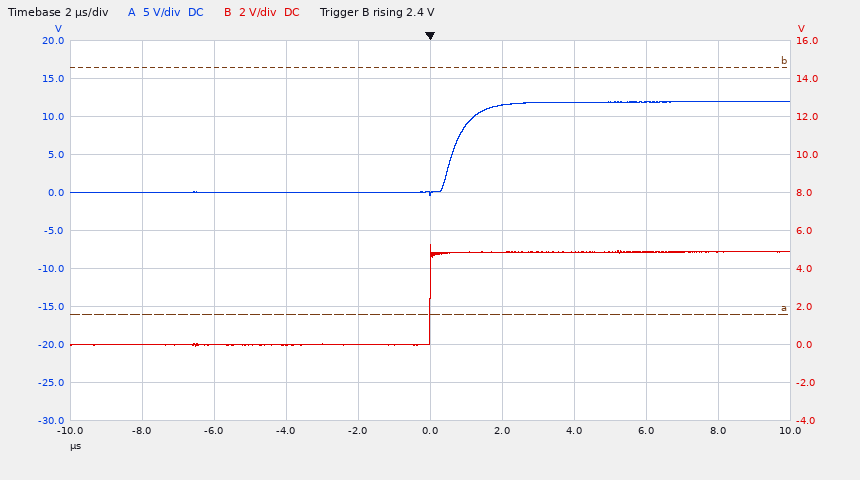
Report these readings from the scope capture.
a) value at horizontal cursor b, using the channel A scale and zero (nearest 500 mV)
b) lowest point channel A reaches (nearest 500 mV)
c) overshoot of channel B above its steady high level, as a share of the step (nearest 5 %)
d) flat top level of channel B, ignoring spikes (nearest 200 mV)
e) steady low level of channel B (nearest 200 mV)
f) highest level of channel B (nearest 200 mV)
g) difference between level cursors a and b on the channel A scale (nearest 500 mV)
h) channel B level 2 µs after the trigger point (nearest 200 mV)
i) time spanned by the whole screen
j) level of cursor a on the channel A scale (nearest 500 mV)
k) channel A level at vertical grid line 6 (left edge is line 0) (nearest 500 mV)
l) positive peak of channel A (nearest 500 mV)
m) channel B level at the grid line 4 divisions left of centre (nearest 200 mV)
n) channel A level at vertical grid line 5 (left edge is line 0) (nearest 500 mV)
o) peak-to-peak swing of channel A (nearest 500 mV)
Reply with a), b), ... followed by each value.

a) 16.5 V
b) -500 mV
c) 10 %
d) 4.8 V
e) 0.0 V
f) 5.2 V
g) 32.5 V
h) 4.8 V
i) 20 µs
j) -16.0 V
k) 11.5 V
l) 12.0 V
m) 0.0 V
n) 0.0 V
o) 12.5 V
